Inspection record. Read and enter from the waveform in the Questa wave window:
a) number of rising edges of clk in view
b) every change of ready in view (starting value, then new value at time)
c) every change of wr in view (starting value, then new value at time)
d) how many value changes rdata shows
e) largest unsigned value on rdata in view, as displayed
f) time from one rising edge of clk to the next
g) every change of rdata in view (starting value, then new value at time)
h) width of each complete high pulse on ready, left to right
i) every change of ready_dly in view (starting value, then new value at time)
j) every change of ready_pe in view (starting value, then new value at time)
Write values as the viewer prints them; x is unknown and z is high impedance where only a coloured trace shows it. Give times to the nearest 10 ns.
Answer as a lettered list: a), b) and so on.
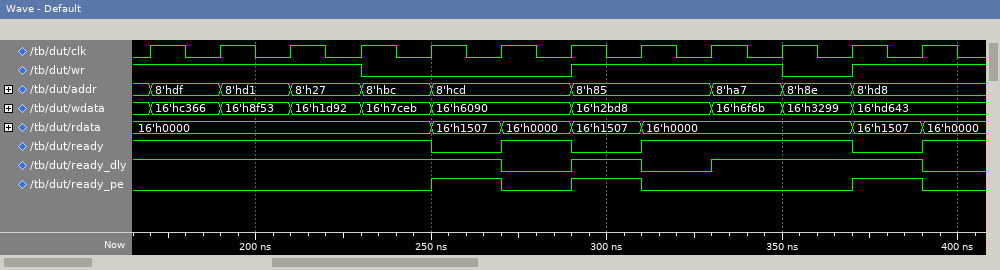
a) 12
b) 1, 0 at 250 ns, 1 at 270 ns, 0 at 290 ns, 1 at 310 ns, 0 at 370 ns, 1 at 390 ns
c) 1, 0 at 230 ns, 1 at 290 ns, 0 at 350 ns, 1 at 370 ns
d) 6
e) 16'h1507
f) 20 ns
g) 16'h0000, 16'h1507 at 250 ns, 16'h0000 at 270 ns, 16'h1507 at 290 ns, 16'h0000 at 310 ns, 16'h1507 at 370 ns, 16'h0000 at 390 ns
h) 20 ns, 60 ns
i) 1, 0 at 270 ns, 1 at 290 ns, 0 at 310 ns, 1 at 330 ns, 0 at 390 ns
j) 0, 1 at 250 ns, 0 at 270 ns, 1 at 290 ns, 0 at 310 ns, 1 at 370 ns, 0 at 390 ns
